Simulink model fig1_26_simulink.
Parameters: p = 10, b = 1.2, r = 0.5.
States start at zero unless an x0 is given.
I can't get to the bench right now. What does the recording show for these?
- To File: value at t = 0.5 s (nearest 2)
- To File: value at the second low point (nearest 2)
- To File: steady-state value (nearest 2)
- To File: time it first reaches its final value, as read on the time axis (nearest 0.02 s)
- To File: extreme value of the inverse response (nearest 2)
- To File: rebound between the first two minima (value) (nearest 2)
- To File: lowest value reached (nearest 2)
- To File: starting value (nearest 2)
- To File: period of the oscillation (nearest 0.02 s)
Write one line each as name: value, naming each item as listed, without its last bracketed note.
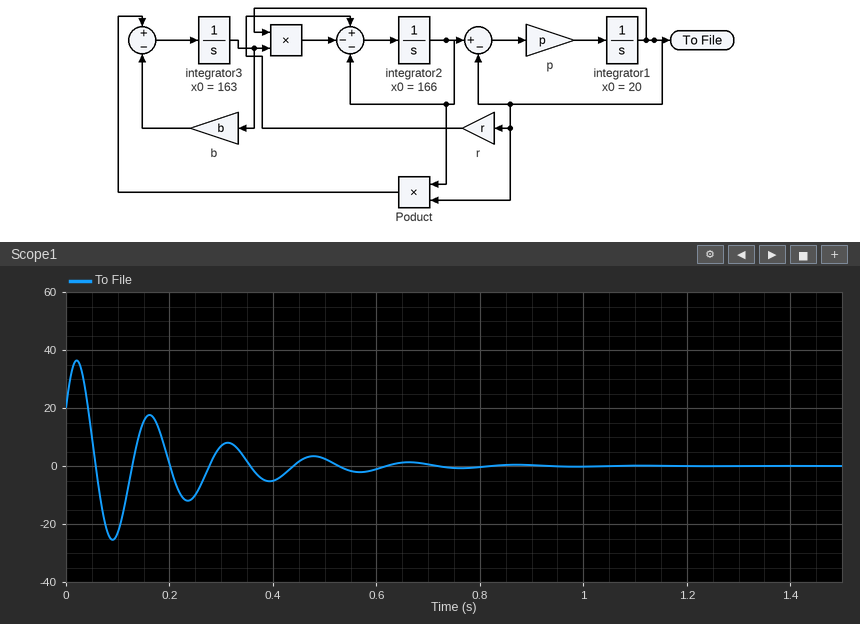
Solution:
To File: value at t = 0.5 s: 2
To File: value at the second low point: -12
To File: steady-state value: 0
To File: time it first reaches its final value, as read on the time axis: 0.06 s
To File: extreme value of the inverse response: 36
To File: rebound between the first two minima (value): 18
To File: lowest value reached: -26
To File: starting value: 20
To File: period of the oscillation: 0.14 s
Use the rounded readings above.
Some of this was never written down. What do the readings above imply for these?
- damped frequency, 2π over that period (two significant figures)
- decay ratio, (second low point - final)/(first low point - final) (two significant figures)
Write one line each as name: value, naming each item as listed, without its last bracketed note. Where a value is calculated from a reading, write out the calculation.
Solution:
damped frequency, 2π over that period: 2π / 0.14 = 45 rad/s
decay ratio, (second low point - final)/(first low point - final): (-12 - 0) / (-26 - 0) = 0.46
